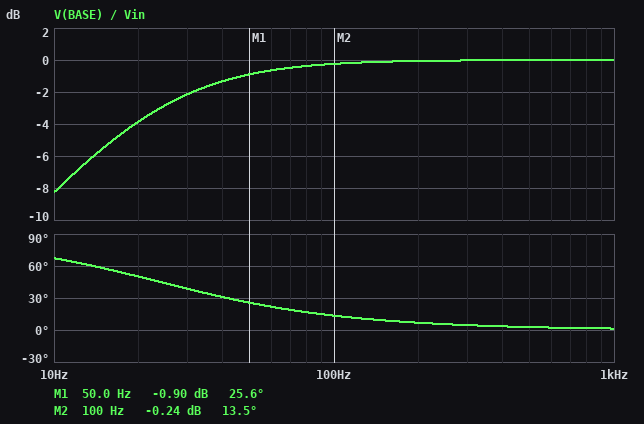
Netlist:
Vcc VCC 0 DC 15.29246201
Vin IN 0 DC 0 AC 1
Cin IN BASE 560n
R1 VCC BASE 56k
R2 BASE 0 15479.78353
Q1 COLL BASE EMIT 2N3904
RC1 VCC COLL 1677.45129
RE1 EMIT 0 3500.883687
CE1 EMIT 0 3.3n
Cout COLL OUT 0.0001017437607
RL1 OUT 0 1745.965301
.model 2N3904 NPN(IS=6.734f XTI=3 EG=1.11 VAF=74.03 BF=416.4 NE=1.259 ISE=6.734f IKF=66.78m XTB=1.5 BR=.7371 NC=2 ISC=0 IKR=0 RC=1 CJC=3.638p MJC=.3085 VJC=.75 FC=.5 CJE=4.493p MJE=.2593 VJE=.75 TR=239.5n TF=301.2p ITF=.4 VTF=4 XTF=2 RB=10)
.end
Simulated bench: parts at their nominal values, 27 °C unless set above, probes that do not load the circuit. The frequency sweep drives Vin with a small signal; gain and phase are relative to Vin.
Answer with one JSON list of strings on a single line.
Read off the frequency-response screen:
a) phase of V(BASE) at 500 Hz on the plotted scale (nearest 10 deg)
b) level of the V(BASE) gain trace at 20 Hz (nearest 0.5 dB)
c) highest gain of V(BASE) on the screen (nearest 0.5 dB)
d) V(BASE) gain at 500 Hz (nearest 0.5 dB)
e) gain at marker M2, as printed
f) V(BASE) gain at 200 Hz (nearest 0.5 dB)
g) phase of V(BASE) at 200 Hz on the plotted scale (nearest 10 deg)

["0 deg", "-4.0 dB", "0 dB", "0 dB", "-0.24 dB", "0 dB", "10 deg"]
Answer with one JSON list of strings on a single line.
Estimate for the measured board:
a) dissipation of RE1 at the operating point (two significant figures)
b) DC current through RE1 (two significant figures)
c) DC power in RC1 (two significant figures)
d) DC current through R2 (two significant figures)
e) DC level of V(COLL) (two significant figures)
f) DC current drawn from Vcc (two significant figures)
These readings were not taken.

["1.9 mW", "740 µA", "910 µW", "210 µA", "14 V", "950 µA"]
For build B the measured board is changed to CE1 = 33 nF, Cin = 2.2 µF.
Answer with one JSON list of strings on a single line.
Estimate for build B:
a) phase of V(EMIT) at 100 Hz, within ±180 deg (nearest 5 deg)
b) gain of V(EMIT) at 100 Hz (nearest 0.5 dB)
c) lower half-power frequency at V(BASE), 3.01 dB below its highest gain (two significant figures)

["5 deg", "0 dB", "6.1 Hz"]
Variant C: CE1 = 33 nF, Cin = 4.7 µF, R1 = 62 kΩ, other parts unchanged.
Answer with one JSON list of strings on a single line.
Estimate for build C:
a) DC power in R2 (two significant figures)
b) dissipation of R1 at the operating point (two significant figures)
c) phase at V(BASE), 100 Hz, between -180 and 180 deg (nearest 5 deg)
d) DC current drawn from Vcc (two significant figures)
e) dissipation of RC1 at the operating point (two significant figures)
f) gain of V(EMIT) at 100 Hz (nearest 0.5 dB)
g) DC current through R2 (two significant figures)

["580 µW", "2.4 mW", "0 deg", "860 µA", "740 µW", "0 dB", "190 µA"]
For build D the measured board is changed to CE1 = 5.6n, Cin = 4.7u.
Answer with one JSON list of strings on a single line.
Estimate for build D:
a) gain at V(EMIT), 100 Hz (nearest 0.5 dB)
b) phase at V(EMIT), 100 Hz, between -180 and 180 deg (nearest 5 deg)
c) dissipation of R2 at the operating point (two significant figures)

["0 dB", "0 deg", "680 µW"]
